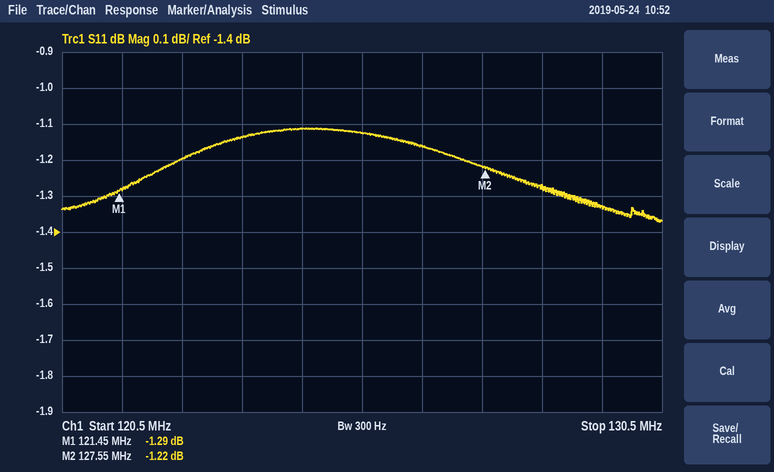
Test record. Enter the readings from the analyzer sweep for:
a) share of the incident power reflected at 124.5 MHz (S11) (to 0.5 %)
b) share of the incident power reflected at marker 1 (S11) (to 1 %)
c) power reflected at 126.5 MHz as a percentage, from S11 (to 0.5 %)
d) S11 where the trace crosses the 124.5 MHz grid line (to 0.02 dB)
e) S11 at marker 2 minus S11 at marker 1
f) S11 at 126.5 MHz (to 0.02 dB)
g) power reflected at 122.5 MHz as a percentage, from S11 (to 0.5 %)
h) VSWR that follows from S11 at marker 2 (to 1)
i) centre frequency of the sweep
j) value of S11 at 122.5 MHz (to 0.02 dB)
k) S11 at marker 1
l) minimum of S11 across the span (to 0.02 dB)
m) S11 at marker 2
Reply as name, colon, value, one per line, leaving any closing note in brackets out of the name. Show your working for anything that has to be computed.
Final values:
share of the incident power reflected at 124.5 MHz (S11): 10^(-1.12/10) ≈ 77.3 %, so 77.5 % to the nearest 0.5 %
share of the incident power reflected at marker 1 (S11): 10^(-1.29/10) ≈ 74 %
power reflected at 126.5 MHz as a percentage, from S11: 10^(-1.16/10) ≈ 76.6 %, so 76.5 % to the nearest 0.5 %
S11 where the trace crosses the 124.5 MHz grid line: -1.12 dB
S11 at marker 2 minus S11 at marker 1: -1.22 − (-1.29) = 0.07 dB
S11 at 126.5 MHz: -1.16 dB
power reflected at 122.5 MHz as a percentage, from S11: 10^(-1.2/10) ≈ 75.9 %, so 76.0 % to the nearest 0.5 %
VSWR that follows from S11 at marker 2: (1 + 0.8690)/(1 − 0.8690) ≈ 14
centre frequency of the sweep: 125.5 MHz
value of S11 at 122.5 MHz: -1.20 dB
S11 at marker 1: -1.29 dB
minimum of S11 across the span: -1.38 dB
S11 at marker 2: -1.22 dB
